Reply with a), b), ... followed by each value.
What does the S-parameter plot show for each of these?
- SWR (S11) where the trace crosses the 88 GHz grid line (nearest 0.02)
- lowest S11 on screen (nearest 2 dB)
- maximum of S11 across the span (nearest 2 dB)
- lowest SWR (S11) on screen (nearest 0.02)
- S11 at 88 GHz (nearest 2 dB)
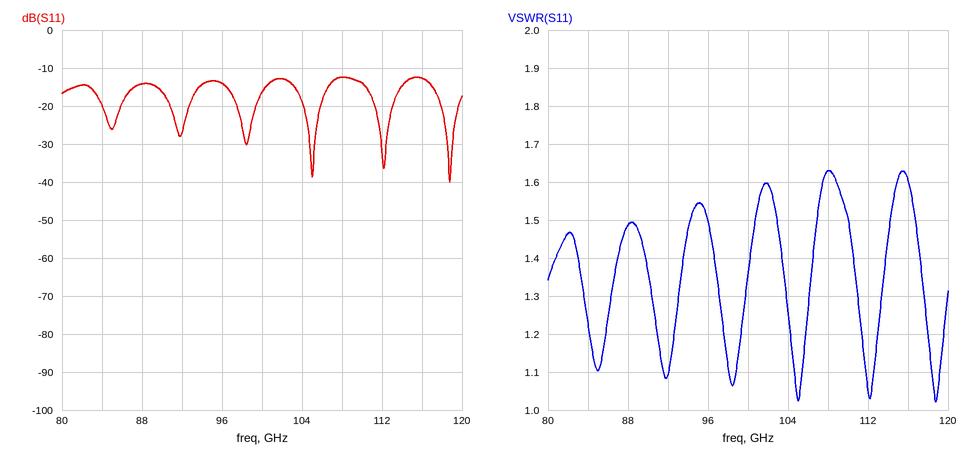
a) 1.48
b) -40 dB
c) -12 dB
d) 1.02
e) -14 dB
